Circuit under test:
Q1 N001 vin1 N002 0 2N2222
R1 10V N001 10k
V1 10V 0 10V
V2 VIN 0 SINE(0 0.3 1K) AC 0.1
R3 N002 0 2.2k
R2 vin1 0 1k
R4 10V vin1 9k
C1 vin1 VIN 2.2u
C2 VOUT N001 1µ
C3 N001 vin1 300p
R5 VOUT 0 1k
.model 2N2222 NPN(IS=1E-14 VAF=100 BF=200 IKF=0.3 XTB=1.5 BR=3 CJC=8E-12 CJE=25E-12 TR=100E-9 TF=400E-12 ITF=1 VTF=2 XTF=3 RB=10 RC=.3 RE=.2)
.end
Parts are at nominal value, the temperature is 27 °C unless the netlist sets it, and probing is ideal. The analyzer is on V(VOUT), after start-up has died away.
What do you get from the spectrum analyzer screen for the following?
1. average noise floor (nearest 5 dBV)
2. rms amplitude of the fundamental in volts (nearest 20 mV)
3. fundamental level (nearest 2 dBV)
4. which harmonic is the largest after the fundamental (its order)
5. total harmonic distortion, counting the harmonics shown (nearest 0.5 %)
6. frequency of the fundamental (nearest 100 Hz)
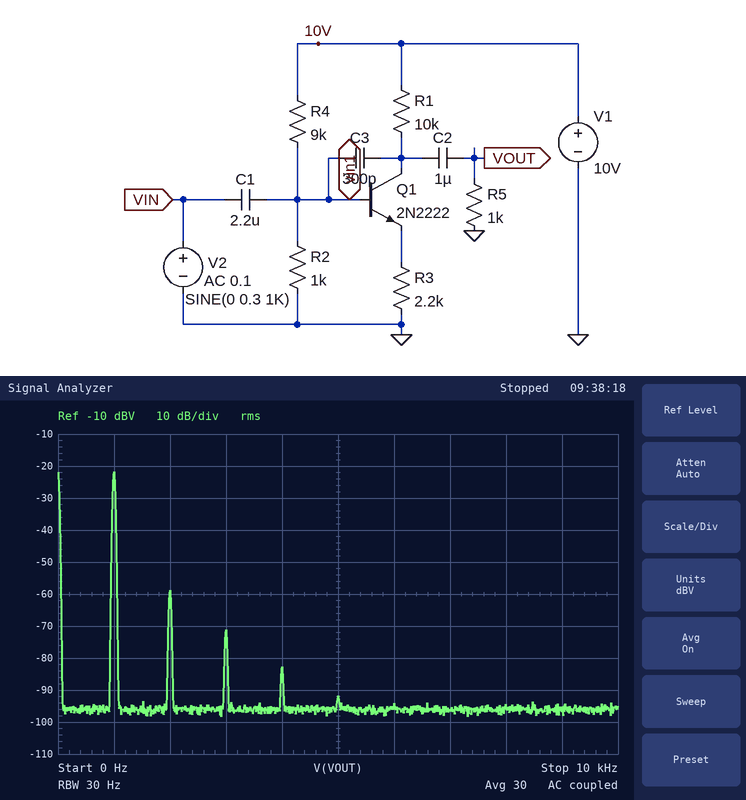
-95 dBV
80 mV
-22 dBV
2
1.5 %
1.0 kHz
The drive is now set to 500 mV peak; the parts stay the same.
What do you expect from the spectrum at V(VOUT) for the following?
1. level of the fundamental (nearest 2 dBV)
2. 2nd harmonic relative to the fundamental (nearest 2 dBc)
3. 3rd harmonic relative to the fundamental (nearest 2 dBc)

-18 dBV
-26 dBc
-32 dBc
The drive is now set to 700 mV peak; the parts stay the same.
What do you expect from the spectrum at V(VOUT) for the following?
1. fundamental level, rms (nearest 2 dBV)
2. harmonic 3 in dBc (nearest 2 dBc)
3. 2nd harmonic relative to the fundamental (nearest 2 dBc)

-16 dBV
-24 dBc
-18 dBc
